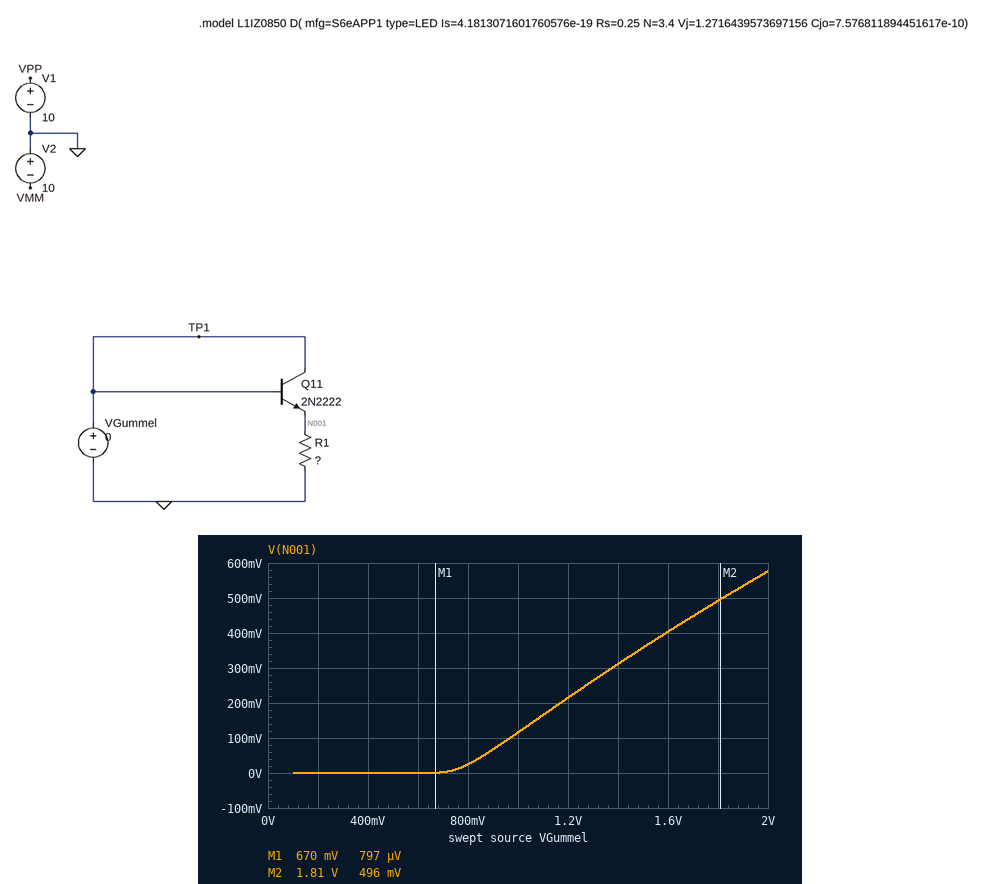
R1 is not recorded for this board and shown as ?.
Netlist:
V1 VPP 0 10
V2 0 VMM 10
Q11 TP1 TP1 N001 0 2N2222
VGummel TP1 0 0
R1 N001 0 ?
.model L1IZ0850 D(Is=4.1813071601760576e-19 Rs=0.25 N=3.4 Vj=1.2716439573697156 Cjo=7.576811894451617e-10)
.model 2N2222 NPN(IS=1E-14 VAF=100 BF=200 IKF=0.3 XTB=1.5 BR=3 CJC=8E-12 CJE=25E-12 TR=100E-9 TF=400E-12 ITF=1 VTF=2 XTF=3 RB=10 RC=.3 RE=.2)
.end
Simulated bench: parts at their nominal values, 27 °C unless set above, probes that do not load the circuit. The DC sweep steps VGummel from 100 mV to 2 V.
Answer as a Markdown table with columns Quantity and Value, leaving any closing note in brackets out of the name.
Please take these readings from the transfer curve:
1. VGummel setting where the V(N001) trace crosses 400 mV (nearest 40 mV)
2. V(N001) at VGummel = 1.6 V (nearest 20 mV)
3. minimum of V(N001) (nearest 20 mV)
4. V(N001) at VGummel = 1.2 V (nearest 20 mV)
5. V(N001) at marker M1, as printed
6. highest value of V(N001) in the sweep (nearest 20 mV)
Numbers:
| Quantity | Value |
|---|---|
| VGummel setting where the V(N001) trace crosses 400 mV | 1.60 V |
| V(N001) at VGummel = 1.6 V | 400 mV |
| minimum of V(N001) | 0 V |
| V(N001) at VGummel = 1.2 V | 220 mV |
| V(N001) at marker M1, as printed | 797 µV |
| highest value of V(N001) in the sweep | 580 mV |
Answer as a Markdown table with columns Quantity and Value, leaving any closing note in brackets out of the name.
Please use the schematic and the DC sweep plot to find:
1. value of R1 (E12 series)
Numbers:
| Quantity | Value |
|---|---|
| value of R1 | 0.47 Ω |
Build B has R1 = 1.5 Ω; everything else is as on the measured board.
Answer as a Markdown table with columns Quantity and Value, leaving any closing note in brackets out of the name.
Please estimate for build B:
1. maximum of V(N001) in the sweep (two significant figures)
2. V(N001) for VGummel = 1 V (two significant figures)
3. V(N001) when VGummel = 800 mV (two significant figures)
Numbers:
| Quantity | Value |
|---|---|
| maximum of V(N001) in the sweep | 930 mV |
| V(N001) for VGummel = 1 V | 180 mV |
| V(N001) when VGummel = 800 mV | 46 mV |
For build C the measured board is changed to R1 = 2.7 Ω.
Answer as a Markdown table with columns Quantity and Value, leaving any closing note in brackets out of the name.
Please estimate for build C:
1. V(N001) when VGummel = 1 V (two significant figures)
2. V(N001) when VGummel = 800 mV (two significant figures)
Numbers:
| Quantity | Value |
|---|---|
| V(N001) when VGummel = 1 V | 210 mV |
| V(N001) when VGummel = 800 mV | 58 mV |
